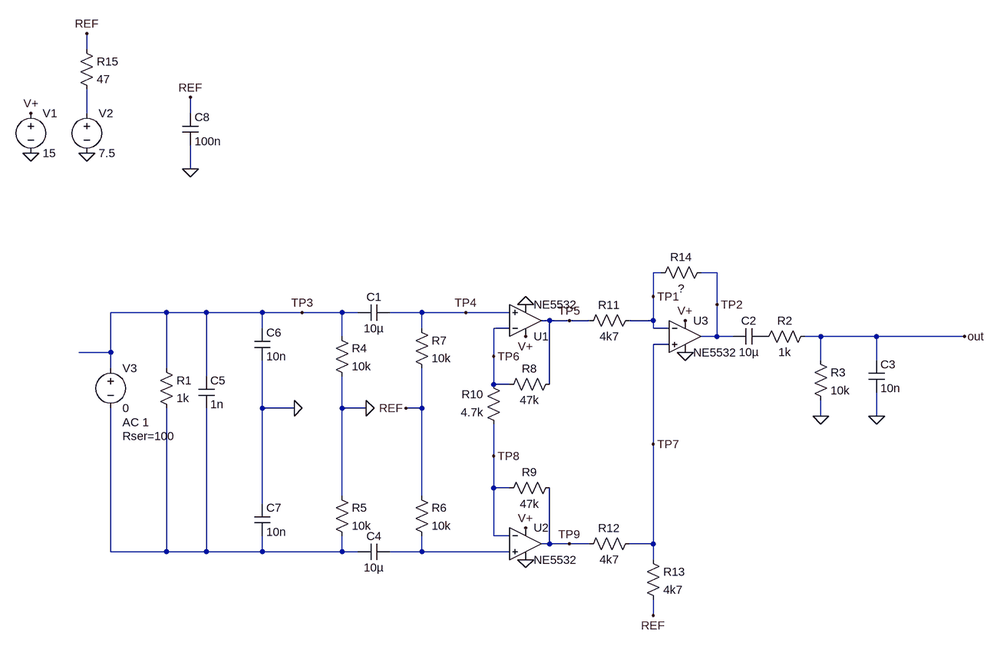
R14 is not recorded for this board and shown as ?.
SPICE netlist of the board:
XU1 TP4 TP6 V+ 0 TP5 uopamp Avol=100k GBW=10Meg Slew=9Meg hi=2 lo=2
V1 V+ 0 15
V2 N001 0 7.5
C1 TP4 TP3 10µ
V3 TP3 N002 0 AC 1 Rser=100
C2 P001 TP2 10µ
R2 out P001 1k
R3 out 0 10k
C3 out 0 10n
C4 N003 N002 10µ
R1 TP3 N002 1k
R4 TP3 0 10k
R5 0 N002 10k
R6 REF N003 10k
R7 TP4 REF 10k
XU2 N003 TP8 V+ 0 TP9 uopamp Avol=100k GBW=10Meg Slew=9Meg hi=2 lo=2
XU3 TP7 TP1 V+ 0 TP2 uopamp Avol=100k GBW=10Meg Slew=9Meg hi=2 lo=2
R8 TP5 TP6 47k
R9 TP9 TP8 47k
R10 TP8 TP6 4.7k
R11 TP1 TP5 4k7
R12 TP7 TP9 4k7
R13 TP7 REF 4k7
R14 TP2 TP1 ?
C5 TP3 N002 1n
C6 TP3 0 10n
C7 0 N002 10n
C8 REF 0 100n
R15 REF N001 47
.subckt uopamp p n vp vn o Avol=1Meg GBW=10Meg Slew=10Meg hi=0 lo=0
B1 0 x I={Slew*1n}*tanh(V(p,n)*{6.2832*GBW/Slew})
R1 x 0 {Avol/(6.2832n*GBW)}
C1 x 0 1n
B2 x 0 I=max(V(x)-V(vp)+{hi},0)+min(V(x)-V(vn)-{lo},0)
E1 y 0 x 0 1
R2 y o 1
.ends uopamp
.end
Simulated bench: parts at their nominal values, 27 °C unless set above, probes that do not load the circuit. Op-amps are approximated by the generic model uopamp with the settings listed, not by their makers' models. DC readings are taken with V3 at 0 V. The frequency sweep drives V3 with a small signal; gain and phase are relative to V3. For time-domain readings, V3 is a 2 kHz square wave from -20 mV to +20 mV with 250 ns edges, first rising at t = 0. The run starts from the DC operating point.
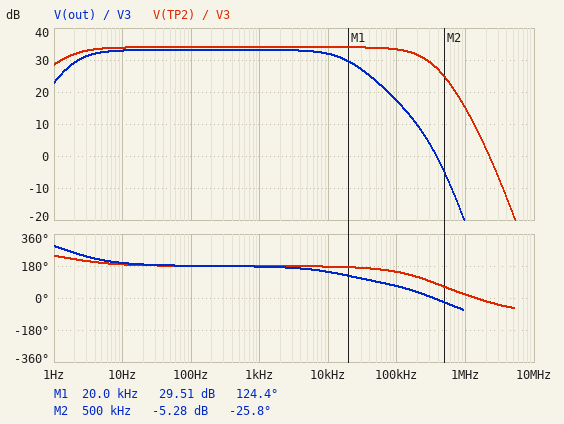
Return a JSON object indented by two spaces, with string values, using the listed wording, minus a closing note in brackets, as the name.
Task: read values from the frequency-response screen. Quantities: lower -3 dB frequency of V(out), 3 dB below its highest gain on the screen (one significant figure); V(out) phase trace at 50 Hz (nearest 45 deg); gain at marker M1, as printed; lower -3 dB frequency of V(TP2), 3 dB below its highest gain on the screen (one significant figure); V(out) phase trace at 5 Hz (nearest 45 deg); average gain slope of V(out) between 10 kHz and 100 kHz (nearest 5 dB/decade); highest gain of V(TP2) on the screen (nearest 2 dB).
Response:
{
  "lower -3 dB frequency of V(out), 3 dB below its highest gain on the screen": "2 Hz",
  "V(out) phase trace at 50 Hz": "180 deg",
  "gain at marker M1, as printed": "29.51 dB",
  "lower -3 dB frequency of V(TP2), 3 dB below its highest gain on the screen": "2 Hz",
  "V(out) phase trace at 5 Hz": "225 deg",
  "average gain slope of V(out) between 10 kHz and 100 kHz": "-15 dB/decade",
  "highest gain of V(TP2) on the screen": "34 dB"
}
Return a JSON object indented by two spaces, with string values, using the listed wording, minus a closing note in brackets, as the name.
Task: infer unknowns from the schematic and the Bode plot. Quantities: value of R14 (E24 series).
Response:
{
  "value of R14": "15 kΩ"
}
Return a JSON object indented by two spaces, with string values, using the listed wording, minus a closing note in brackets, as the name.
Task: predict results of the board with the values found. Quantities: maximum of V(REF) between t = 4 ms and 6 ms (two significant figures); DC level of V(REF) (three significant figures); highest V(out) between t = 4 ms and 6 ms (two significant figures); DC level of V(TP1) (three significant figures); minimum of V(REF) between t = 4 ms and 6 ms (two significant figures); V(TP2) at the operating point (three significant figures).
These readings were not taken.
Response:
{
  "maximum of V(REF) between t = 4 ms and 6 ms": "7.5 V",
  "DC level of V(REF)": "7.50 V",
  "highest V(out) between t = 4 ms and 6 ms": "100 mV",
  "DC level of V(TP1)": "7.50 V",
  "minimum of V(REF) between t = 4 ms and 6 ms": "7.5 V",
  "V(TP2) at the operating point": "7.50 V"
}
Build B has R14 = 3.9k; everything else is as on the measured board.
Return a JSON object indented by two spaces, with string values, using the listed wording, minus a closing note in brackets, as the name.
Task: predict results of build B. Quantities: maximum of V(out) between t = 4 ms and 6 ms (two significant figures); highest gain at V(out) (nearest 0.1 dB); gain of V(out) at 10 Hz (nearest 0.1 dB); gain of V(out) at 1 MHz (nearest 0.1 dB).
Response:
{
  "maximum of V(out) between t = 4 ms and 6 ms": "33 mV",
  "highest gain at V(out)": "23.5 dB",
  "gain of V(out) at 10 Hz": "23.3 dB",
  "gain of V(out) at 1 MHz": "-30.1 dB"
}
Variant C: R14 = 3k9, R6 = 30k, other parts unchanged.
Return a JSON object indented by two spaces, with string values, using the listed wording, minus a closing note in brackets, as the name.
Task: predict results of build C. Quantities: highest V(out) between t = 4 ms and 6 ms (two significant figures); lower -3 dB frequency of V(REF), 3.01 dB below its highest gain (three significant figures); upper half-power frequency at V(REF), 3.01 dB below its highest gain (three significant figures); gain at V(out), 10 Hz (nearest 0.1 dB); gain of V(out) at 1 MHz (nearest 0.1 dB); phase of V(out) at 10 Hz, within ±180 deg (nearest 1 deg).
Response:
{
  "highest V(out) between t = 4 ms and 6 ms": "27 mV",
  "lower -3 dB frequency of V(REF), 3.01 dB below its highest gain": "999 mHz",
  "upper half-power frequency at V(REF), 3.01 dB below its highest gain": "31.9 kHz",
  "gain at V(out), 10 Hz": "23.4 dB",
  "gain of V(out) at 1 MHz": "-30.1 dB",
  "phase of V(out) at 10 Hz, within ±180 deg": "-166 deg"
}
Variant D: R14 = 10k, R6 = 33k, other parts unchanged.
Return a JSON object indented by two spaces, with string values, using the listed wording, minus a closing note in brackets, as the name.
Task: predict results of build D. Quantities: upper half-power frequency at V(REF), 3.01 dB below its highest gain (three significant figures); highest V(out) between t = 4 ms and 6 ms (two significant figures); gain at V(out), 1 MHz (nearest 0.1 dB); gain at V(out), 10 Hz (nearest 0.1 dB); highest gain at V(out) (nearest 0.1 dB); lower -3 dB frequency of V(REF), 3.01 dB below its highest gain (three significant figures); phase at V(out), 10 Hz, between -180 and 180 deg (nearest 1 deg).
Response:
{
  "upper half-power frequency at V(REF), 3.01 dB below its highest gain": "31.8 kHz",
  "highest V(out) between t = 4 ms and 6 ms": "56 mV",
  "gain at V(out), 1 MHz": "-23.8 dB",
  "gain at V(out), 10 Hz": "29.9 dB",
  "highest gain at V(out)": "30.0 dB",
  "lower -3 dB frequency of V(REF), 3.01 dB below its highest gain": "970 mHz",
  "phase at V(out), 10 Hz, between -180 and 180 deg": "-166 deg"
}
